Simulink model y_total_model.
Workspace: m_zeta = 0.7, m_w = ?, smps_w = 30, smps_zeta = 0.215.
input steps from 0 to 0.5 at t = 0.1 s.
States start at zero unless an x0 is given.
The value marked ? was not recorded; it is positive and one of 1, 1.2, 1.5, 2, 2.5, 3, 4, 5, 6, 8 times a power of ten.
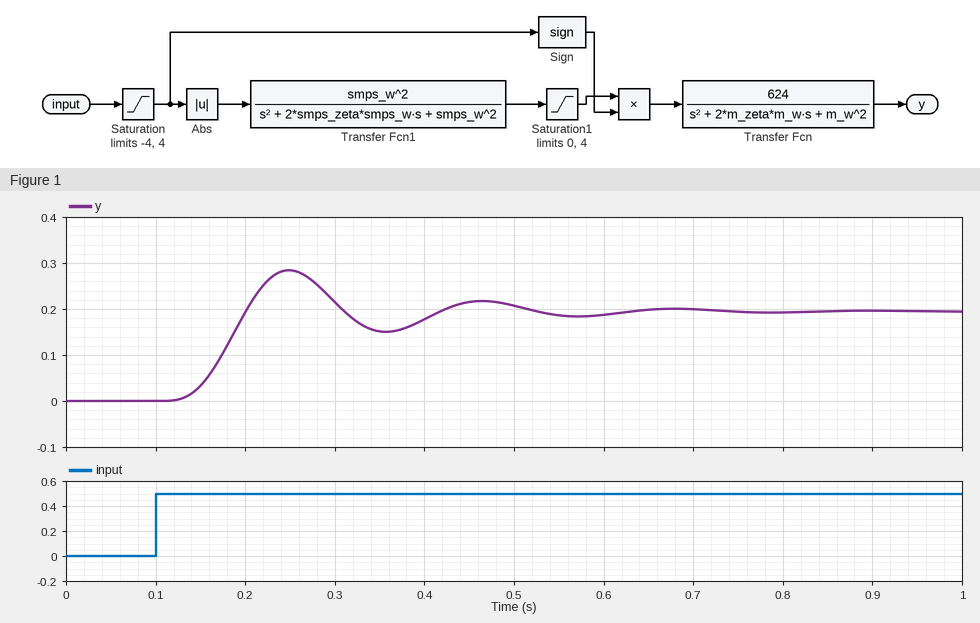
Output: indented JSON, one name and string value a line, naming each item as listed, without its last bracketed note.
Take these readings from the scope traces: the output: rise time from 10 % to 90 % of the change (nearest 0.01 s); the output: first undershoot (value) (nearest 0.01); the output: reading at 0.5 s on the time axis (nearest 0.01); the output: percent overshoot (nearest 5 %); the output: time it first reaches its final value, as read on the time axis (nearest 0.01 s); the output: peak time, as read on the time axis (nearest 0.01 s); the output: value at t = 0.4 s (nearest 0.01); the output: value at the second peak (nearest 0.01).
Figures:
{
  "the output: rise time from 10 % to 90 % of the change": "0.05 s",
  "the output: first undershoot (value)": "0.15",
  "the output: reading at 0.5 s on the time axis": "0.21",
  "the output: percent overshoot": "45 %",
  "the output: time it first reaches its final value, as read on the time axis": "0.20 s",
  "the output: peak time, as read on the time axis": "0.25 s",
  "the output: value at t = 0.4 s": "0.18",
  "the output: value at the second peak": "0.22"
}
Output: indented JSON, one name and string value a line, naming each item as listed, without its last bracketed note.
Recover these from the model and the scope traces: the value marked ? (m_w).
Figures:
{
  "the value marked ?": "40"
}
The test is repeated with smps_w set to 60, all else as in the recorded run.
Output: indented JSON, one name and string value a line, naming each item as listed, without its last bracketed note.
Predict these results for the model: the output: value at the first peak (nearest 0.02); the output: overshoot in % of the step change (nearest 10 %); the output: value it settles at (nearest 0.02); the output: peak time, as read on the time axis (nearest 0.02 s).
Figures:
{
  "the output: value at the first peak": "0.24",
  "the output: overshoot in % of the step change": "20 %",
  "the output: value it settles at": "0.20",
  "the output: peak time, as read on the time axis": "0.20 s"
}
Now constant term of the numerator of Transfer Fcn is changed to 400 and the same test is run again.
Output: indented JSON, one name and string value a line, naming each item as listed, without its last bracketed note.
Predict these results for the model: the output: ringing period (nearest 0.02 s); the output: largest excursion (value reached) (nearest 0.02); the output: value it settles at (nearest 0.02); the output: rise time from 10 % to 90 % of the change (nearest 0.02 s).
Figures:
{
  "the output: ringing period": "0.22 s",
  "the output: largest excursion (value reached)": "0.18",
  "the output: value it settles at": "0.12",
  "the output: rise time from 10 % to 90 % of the change": "0.06 s"
}
